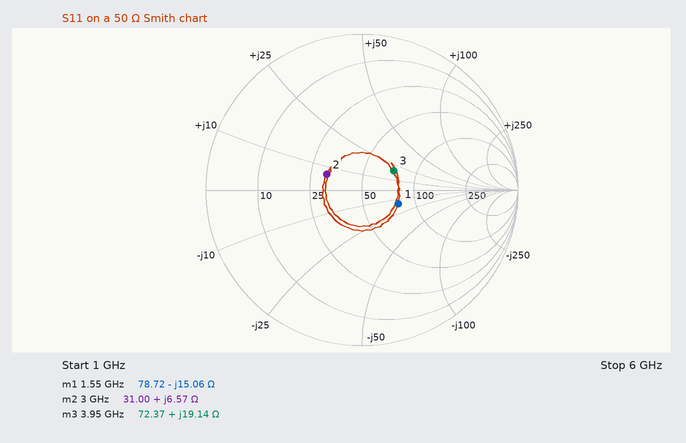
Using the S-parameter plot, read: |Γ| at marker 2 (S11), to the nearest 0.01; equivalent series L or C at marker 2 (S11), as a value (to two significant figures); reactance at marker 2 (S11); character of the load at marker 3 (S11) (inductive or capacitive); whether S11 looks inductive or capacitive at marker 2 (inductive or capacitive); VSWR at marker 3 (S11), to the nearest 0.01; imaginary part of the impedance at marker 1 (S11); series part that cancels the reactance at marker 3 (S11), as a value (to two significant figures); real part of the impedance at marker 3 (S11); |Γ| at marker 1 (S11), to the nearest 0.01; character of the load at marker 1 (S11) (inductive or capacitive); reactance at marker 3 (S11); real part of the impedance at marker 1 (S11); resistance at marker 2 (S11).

0.25
350 pH
+6.57 Ω
inductive
inductive
1.62
-15.06 Ω
2.1 pF
72.37 Ω
0.25
capacitive
+19.14 Ω
78.72 Ω
31.00 Ω
